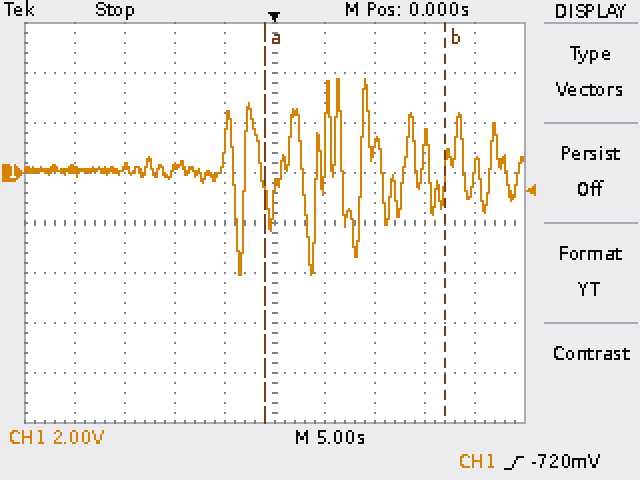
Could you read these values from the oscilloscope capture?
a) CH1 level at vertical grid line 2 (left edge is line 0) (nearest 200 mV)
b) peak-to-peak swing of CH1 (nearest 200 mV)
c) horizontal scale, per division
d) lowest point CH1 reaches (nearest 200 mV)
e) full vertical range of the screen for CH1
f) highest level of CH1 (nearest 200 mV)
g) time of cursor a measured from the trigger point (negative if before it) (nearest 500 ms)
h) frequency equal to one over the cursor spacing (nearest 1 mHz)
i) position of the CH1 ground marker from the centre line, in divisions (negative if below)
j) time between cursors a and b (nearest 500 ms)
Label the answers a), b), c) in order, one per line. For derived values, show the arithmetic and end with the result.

a) 200 mV
b) 3.8 V − (-4.0 V) = 7.8 V
c) 5 s
d) -4.0 V
e) 16 V
f) 3.8 V
g) -1.0 s
h) 1 / 18.0 s ≈ 56 mHz
i) +1.0 div
j) 18.0 s
